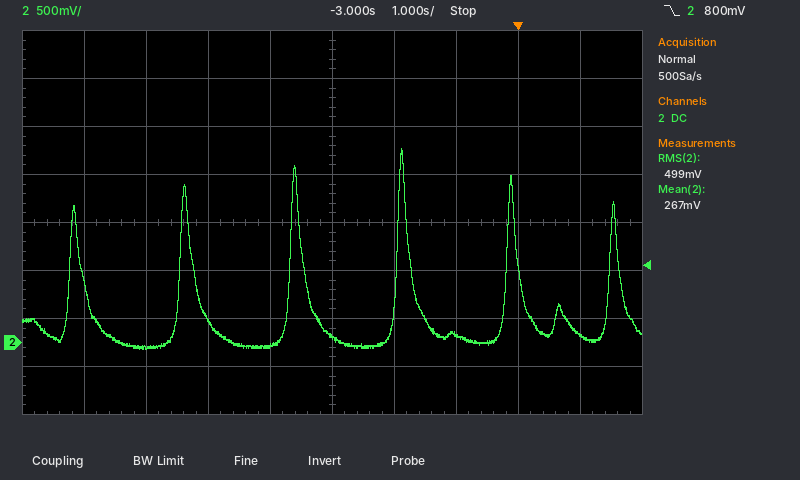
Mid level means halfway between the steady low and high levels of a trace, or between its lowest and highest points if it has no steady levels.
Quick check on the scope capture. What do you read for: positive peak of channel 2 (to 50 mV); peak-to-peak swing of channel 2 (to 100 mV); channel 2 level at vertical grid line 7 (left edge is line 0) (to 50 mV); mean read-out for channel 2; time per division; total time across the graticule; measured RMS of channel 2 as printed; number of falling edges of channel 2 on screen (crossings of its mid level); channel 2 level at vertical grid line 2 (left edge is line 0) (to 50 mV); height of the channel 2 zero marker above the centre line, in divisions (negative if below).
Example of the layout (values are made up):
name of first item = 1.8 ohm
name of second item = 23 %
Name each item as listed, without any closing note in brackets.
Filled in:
positive peak of channel 2 = 2.00 V
peak-to-peak swing of channel 2 = 2.10 V
channel 2 level at vertical grid line 7 (left edge is line 0) = 100 mV
mean read-out for channel 2 = 267 mV
time per division = 1 s
total time across the graticule = 10 s
measured RMS of channel 2 as printed = 499 mV
number of falling edges of channel 2 on screen = 6
channel 2 level at vertical grid line 2 (left edge is line 0) = -50 mV
height of the channel 2 zero marker above the centre line, in divisions = -2.5 div
